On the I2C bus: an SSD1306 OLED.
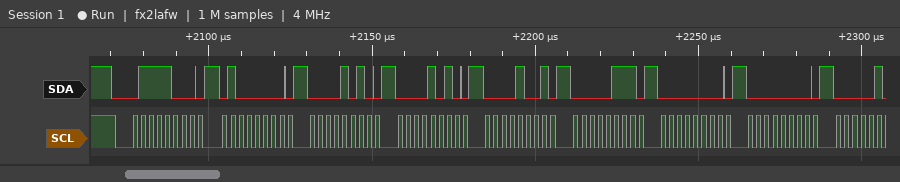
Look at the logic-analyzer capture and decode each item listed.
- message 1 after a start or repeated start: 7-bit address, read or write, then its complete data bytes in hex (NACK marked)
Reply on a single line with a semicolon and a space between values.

0x3C write: 40 0A 0A 09 07 00 00
